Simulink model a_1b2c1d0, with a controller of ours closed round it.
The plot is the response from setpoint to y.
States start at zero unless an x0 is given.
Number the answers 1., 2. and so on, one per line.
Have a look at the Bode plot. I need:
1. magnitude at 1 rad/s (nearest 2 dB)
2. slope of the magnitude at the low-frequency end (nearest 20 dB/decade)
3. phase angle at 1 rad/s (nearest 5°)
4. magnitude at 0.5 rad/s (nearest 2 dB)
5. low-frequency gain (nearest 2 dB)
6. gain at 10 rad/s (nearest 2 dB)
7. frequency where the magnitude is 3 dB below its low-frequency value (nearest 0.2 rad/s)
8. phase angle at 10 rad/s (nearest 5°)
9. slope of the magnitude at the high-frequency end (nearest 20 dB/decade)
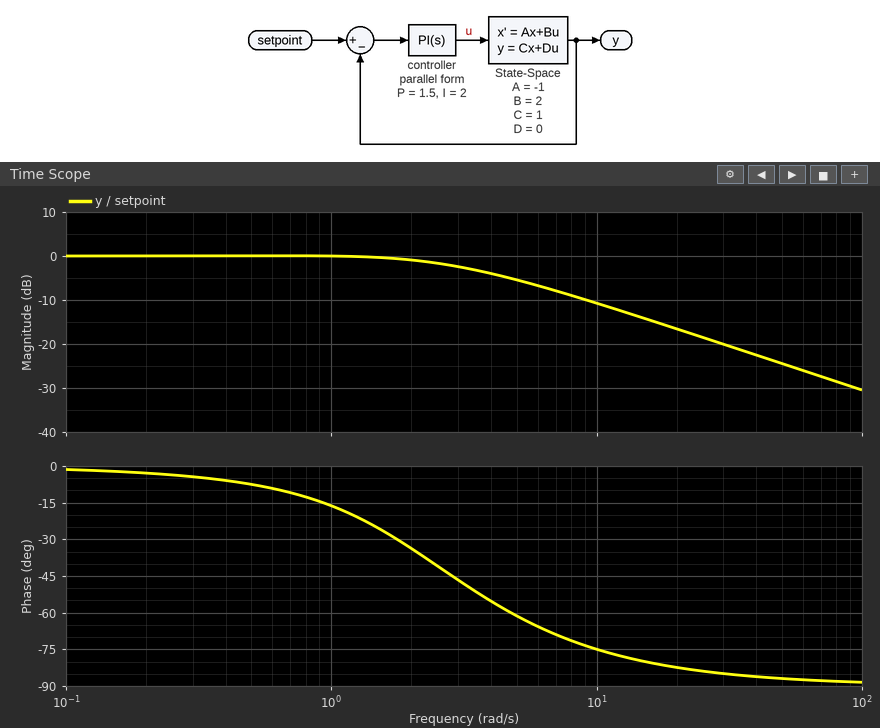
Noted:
1. 0 dB
2. 0 dB/decade
3. -15°
4. 0 dB
5. 0 dB
6. -10 dB
7. 3.4 rad/s
8. -75°
9. -20 dB/decade
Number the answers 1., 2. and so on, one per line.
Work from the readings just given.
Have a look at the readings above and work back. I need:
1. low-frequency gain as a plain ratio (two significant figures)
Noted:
1. 1.0
